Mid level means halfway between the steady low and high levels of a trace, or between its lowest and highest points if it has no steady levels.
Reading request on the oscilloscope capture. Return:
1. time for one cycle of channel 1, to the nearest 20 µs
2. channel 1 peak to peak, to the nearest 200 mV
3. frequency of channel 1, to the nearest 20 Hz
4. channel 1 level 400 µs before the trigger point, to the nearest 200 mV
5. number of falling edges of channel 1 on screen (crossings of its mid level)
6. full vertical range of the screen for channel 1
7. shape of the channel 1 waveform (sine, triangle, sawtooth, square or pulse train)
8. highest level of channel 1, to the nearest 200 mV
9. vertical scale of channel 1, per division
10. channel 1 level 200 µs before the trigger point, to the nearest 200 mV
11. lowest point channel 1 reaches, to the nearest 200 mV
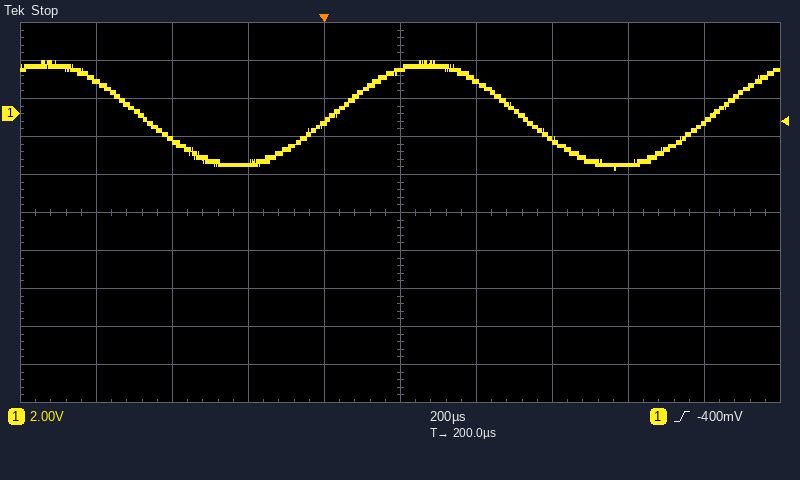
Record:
1.00 ms
5.8 V
1.00 kHz
-1.4 V
2
20 V
sine
2.8 V
2 V
-2.6 V
-3.0 V
